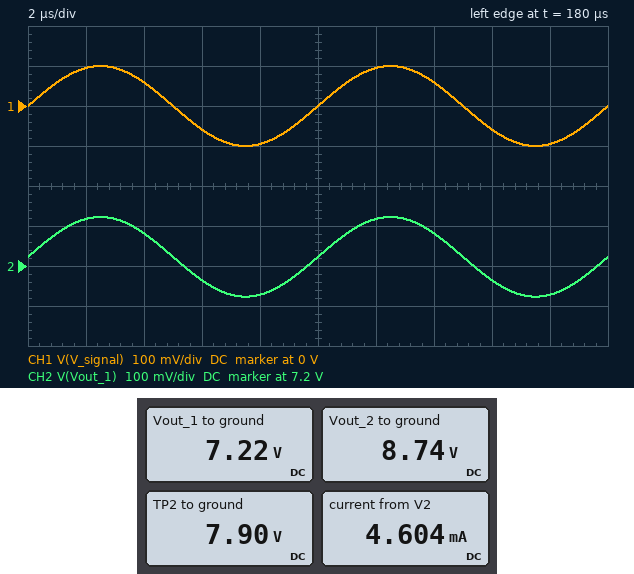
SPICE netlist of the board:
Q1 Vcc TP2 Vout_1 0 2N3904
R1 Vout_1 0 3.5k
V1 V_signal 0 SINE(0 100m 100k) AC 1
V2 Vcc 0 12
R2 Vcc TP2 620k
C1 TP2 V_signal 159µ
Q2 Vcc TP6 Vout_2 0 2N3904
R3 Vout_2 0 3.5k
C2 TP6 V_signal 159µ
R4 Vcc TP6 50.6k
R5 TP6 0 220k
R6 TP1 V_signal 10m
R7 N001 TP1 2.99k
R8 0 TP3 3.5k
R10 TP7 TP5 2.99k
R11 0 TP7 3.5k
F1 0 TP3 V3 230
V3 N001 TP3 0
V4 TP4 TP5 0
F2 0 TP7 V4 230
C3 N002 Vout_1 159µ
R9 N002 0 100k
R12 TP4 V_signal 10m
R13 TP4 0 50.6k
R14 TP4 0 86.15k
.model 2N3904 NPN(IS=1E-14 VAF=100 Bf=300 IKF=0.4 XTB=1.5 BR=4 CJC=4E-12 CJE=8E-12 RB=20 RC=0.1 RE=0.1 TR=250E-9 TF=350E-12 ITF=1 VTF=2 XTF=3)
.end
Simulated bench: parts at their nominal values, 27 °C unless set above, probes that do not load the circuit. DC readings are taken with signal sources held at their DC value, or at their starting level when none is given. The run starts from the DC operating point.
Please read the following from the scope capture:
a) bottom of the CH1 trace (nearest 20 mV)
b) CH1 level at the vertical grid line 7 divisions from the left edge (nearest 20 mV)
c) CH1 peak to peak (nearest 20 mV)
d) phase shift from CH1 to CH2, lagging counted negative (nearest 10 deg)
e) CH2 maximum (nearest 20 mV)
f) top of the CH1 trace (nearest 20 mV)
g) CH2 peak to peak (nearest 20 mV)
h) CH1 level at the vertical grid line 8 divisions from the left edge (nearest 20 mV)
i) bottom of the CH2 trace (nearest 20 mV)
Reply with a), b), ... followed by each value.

a) -100 mV
b) 60 mV
c) 200 mV
d) 0 deg
e) 7.32 V
f) 100 mV
g) 200 mV
h) -60 mV
i) 7.12 V
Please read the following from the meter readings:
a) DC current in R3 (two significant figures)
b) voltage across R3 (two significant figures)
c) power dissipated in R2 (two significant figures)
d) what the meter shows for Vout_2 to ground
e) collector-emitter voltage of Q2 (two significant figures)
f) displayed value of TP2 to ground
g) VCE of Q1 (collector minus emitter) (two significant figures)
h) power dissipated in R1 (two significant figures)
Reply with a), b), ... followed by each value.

a) 2.5 mA
b) 8.7 V
c) 27 µW
d) 8.74 V
e) 3.3 V
f) 7.90 V
g) 4.8 V
h) 15 mW
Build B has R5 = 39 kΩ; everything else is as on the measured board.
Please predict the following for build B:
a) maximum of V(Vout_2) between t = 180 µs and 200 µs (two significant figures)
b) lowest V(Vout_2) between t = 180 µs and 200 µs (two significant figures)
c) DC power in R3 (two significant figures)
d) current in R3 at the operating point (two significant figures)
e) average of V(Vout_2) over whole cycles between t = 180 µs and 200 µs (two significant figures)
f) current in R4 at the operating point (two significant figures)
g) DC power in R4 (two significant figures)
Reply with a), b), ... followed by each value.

a) 4.6 V
b) 4.4 V
c) 5.7 mW
d) 1.3 mA
e) 4.5 V
f) 140 µA
g) 930 µW
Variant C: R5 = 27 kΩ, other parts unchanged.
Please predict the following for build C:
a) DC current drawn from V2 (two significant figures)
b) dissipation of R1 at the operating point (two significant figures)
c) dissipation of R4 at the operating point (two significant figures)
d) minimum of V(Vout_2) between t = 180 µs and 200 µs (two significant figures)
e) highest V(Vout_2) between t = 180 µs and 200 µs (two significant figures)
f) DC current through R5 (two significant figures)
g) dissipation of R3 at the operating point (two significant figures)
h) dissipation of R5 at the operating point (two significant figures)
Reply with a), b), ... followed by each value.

a) 3.2 mA
b) 15 mW
c) 1.2 mW
d) 3.4 V
e) 3.6 V
f) 150 µA
g) 3.4 mW
h) 630 µW
